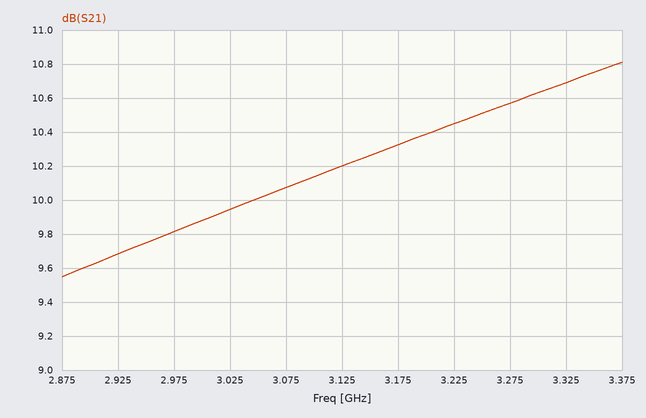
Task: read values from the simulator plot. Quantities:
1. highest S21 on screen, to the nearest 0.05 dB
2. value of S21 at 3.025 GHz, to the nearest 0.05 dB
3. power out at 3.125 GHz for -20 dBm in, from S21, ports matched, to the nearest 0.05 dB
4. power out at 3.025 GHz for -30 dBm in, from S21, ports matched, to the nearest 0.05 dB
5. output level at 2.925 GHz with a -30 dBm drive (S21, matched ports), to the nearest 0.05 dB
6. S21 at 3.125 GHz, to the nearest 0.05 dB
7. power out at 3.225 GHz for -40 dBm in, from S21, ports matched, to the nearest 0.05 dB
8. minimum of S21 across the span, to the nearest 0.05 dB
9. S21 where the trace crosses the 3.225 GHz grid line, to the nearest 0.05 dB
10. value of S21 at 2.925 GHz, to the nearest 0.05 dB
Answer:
10.80 dB
9.95 dB
-9.80 dBm
-20.05 dBm
-20.30 dBm
10.20 dB
-29.55 dBm
9.55 dB
10.45 dB
9.70 dB
